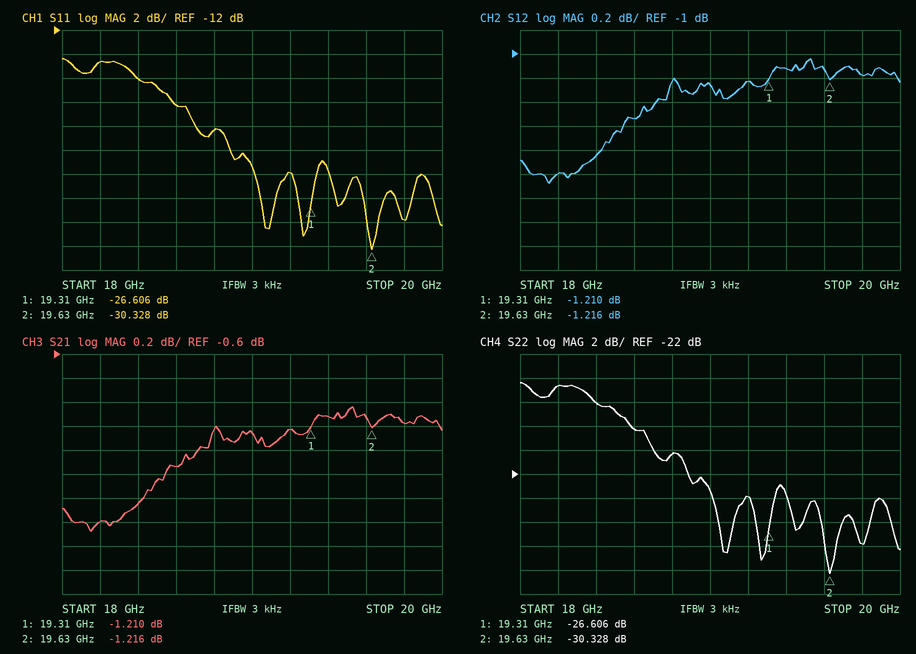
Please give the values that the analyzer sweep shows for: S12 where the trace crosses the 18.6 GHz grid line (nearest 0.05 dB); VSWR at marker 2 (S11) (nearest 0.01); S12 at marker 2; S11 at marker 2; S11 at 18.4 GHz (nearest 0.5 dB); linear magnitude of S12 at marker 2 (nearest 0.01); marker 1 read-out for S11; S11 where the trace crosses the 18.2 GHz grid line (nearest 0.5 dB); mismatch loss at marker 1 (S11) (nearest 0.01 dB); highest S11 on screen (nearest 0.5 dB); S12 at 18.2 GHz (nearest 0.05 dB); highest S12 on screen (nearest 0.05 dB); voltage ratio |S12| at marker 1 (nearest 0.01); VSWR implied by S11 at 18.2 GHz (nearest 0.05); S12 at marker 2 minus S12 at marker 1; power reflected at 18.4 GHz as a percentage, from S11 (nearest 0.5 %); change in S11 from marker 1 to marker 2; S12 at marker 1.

-1.55 dB
1.06
-1.216 dB
-30.328 dB
-16.0 dB
0.87
-26.606 dB
-14.5 dB
0.01 dB
-14.5 dB
-2.00 dB
-1.05 dB
0.87
1.45
-0.006 dB
2.5 %
-3.722 dB
-1.210 dB
